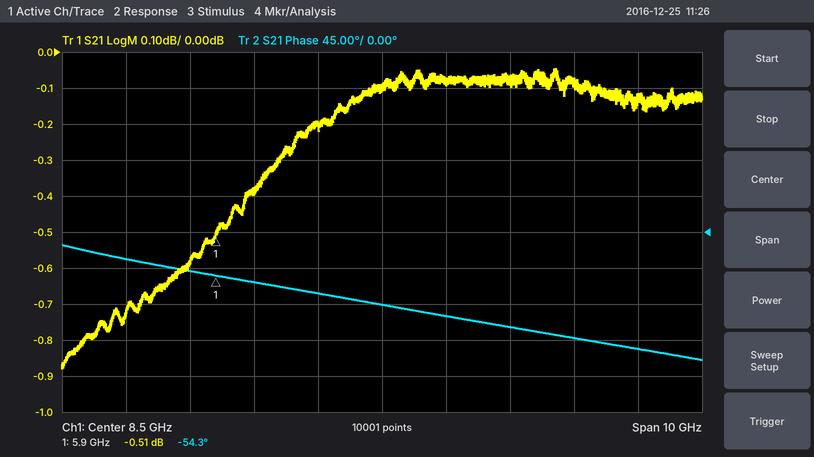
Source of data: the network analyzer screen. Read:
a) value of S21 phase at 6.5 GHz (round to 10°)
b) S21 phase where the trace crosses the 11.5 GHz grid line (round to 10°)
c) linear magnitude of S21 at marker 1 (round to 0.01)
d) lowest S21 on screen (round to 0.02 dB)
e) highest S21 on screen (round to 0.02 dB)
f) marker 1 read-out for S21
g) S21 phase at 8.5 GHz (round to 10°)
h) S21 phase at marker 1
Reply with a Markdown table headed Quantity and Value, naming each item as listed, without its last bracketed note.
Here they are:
| Quantity | Value |
|---|---|
| value of S21 phase at 6.5 GHz | -60° |
| S21 phase where the trace crosses the 11.5 GHz grid line | -130° |
| linear magnitude of S21 at marker 1 | 0.94 |
| lowest S21 on screen | -0.88 dB |
| highest S21 on screen | -0.04 dB |
| marker 1 read-out for S21 | -0.51 dB |
| S21 phase at 8.5 GHz | -90° |
| S21 phase at marker 1 | -54.3° |
